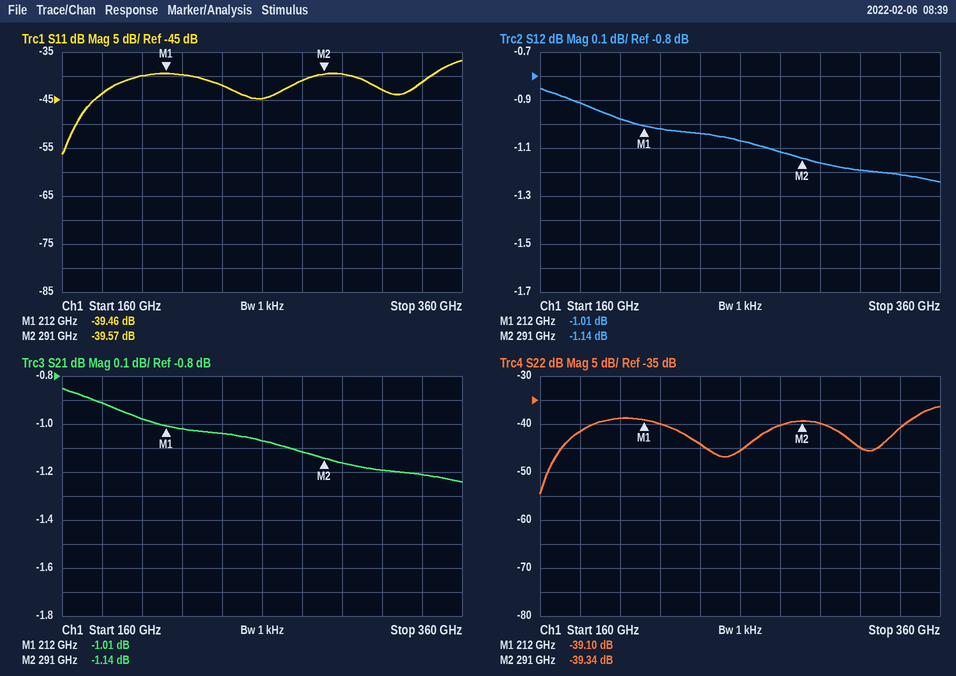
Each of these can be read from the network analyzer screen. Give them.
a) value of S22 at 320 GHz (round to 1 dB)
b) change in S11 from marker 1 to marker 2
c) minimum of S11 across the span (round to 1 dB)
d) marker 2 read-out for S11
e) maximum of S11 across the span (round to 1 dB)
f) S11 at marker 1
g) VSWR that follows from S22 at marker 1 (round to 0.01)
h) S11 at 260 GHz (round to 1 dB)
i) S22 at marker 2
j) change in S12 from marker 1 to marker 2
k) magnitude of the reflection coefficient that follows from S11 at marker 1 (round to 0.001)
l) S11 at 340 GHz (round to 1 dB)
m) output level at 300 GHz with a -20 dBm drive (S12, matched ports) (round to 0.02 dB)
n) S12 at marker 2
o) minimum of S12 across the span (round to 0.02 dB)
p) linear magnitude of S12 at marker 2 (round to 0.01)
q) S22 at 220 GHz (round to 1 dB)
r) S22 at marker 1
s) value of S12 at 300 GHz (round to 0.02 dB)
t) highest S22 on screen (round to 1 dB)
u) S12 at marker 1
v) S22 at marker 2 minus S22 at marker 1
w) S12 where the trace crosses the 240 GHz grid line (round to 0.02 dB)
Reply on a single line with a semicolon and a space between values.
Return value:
-45 dB; -0.11 dB; -56 dB; -39.57 dB; -37 dB; -39.46 dB; 1.02; -45 dB; -39.34 dB; -0.13 dB; 0.011; -41 dB; -21.16 dBm; -1.14 dB; -1.24 dB; 0.88; -40 dB; -39.10 dB; -1.16 dB; -36 dB; -1.01 dB; -0.24 dB; -1.04 dB
